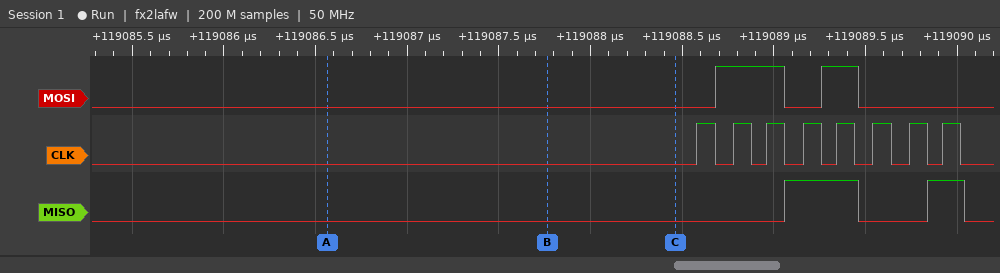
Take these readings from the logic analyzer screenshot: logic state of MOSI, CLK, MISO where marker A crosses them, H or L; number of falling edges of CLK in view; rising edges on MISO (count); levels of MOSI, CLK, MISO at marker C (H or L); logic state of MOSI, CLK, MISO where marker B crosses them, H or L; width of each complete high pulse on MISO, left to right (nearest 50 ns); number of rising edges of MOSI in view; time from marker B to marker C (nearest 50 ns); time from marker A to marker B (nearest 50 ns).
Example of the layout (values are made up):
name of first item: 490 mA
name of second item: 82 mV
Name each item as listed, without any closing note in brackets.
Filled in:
logic state of MOSI, CLK, MISO where marker A crosses them, H or L: MOSI=L, CLK=L, MISO=L
number of falling edges of CLK in view: 8
rising edges on MISO: 2
levels of MOSI, CLK, MISO at marker C: MOSI=L, CLK=L, MISO=L
logic state of MOSI, CLK, MISO where marker B crosses them, H or L: MOSI=L, CLK=L, MISO=L
width of each complete high pulse on MISO, left to right: 400 ns, 200 ns
number of rising edges of MOSI in view: 2
time from marker B to marker C: 700 ns
time from marker A to marker B: 1200 ns
